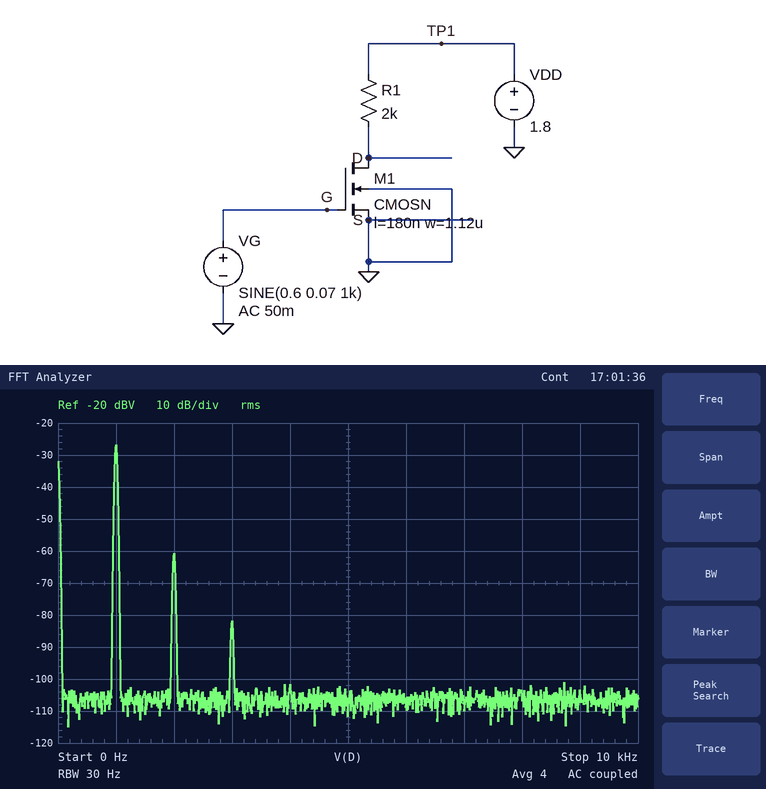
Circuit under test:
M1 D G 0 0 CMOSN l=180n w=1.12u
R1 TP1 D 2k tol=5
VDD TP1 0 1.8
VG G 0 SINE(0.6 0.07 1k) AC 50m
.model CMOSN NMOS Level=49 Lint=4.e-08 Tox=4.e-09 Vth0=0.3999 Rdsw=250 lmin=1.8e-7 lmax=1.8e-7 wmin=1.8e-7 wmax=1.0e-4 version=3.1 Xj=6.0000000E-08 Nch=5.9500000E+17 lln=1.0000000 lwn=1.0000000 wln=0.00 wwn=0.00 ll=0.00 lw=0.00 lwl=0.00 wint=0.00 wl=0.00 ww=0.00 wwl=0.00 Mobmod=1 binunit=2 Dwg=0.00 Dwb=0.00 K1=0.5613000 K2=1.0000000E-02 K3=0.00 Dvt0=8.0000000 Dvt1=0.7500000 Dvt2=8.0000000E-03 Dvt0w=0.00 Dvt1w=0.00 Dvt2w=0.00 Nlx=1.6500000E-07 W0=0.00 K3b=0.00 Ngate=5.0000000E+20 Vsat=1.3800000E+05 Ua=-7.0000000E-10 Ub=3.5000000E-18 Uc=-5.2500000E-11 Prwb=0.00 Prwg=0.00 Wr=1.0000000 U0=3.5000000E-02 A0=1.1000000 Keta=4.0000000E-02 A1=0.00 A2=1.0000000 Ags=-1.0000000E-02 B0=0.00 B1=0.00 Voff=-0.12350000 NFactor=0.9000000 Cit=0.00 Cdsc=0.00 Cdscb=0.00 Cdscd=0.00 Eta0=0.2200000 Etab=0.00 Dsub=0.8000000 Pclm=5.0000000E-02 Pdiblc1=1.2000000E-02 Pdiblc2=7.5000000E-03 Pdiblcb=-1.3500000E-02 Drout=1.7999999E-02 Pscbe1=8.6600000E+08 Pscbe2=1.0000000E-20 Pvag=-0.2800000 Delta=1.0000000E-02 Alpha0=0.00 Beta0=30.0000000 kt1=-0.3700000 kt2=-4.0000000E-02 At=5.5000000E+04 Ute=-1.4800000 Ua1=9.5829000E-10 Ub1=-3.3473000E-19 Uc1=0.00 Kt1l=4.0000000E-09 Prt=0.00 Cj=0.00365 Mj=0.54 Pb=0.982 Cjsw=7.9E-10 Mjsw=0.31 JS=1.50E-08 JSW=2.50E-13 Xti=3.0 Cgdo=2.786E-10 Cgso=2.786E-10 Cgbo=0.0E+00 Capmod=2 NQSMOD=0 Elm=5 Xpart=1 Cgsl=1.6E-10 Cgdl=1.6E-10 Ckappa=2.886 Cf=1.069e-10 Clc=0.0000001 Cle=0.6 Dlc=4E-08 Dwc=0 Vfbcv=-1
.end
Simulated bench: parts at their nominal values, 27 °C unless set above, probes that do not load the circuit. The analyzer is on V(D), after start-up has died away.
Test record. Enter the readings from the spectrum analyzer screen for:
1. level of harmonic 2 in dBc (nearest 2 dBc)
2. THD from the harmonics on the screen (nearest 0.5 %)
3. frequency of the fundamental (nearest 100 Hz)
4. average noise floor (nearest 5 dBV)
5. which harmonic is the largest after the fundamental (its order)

-34 dBc
2.0 %
1.0 kHz
-105 dBV
2
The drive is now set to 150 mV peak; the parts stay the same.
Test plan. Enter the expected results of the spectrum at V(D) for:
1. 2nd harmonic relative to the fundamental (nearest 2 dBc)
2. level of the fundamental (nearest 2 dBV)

-26 dBc
-20 dBV
